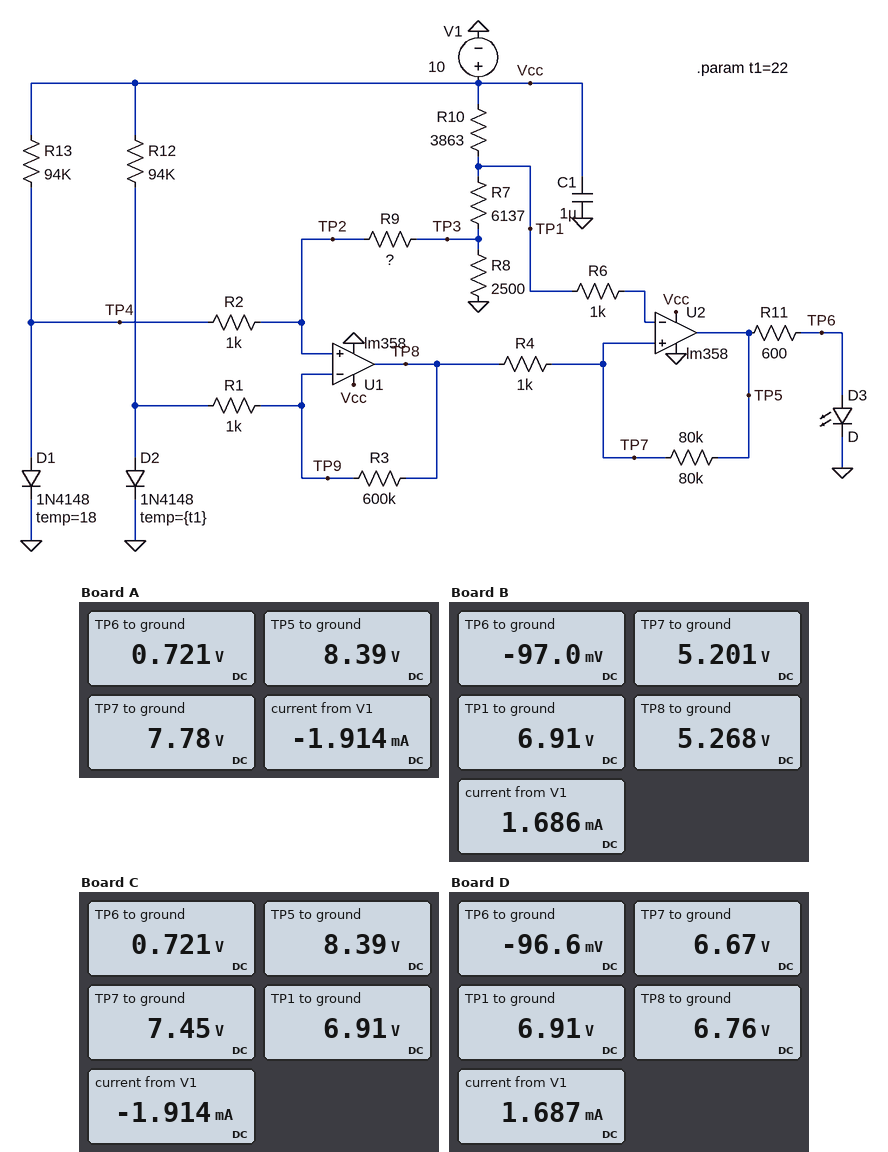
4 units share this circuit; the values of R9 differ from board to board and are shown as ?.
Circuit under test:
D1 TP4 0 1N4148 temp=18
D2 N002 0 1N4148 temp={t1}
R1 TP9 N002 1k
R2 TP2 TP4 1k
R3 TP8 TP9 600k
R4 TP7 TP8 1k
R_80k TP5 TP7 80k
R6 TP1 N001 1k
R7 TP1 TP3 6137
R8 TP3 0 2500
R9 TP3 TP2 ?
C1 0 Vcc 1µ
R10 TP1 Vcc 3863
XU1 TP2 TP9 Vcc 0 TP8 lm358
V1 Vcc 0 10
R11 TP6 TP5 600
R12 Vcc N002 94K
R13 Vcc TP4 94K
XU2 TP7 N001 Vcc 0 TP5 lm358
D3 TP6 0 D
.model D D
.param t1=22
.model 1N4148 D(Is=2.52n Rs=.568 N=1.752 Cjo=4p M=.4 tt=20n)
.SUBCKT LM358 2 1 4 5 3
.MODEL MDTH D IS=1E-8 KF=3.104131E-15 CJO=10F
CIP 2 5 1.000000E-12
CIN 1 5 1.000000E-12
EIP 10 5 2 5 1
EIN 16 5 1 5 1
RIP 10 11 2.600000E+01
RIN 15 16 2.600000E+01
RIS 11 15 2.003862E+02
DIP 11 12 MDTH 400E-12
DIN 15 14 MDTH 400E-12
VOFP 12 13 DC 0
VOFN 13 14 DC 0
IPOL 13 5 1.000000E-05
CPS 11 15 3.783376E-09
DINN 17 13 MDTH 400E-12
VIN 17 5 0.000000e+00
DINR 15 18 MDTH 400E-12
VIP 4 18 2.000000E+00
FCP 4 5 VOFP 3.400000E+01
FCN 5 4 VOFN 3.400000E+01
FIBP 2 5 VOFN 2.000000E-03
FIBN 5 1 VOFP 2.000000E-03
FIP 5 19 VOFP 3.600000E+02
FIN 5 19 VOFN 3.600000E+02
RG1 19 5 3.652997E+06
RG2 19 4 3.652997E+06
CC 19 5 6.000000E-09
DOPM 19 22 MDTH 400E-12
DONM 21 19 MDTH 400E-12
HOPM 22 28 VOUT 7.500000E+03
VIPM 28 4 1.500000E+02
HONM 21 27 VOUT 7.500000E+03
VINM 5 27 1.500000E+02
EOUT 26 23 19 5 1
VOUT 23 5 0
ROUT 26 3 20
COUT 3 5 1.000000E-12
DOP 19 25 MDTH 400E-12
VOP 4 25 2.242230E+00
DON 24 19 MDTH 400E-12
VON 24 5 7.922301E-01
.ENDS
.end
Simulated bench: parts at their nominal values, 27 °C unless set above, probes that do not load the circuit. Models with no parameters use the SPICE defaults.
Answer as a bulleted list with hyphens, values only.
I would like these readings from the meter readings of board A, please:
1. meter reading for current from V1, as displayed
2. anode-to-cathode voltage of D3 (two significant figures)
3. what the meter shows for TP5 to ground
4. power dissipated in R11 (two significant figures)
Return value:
- -1.914 mA
- 720 mV
- 8.39 V
- 98 mW
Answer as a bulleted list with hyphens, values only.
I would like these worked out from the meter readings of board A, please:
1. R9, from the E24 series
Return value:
- 270 kΩ
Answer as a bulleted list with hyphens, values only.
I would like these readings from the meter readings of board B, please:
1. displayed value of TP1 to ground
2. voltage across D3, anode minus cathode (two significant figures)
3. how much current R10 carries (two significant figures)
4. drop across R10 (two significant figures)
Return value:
- 6.91 V
- -97 mV
- 800 µA
- 3.1 V
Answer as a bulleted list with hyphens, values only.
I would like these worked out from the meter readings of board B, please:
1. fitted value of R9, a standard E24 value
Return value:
- 1.1 MΩ
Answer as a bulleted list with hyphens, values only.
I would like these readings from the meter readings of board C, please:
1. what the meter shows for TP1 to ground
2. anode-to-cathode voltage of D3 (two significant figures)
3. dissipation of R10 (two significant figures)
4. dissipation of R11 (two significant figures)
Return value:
- 6.91 V
- 720 mV
- 2.5 mW
- 98 mW
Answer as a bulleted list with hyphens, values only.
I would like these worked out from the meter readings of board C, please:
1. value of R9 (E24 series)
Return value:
- 300 kΩ
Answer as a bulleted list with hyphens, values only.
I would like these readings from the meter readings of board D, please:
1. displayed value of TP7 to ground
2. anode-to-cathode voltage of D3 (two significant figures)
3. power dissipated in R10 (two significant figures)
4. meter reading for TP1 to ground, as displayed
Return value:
- 6.67 V
- -97 mV
- 2.5 mW
- 6.91 V
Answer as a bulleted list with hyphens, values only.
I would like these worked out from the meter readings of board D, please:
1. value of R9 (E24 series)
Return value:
- 390 kΩ
